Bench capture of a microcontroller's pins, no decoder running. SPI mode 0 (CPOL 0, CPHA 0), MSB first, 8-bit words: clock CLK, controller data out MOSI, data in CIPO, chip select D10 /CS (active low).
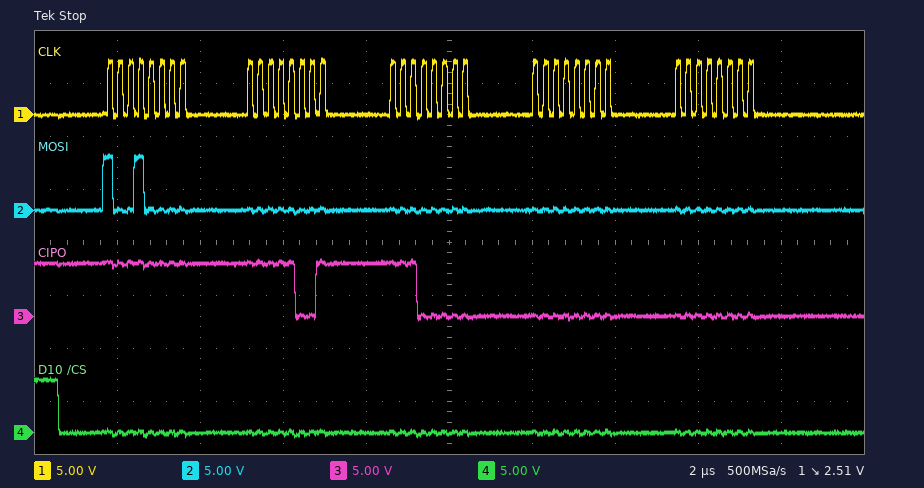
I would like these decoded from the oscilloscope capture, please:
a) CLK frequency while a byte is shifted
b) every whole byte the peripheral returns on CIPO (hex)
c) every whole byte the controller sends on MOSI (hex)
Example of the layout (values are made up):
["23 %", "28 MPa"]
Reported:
["4 MHz", "FF F9 E0 00 00", "90 00 00 00 00"]
